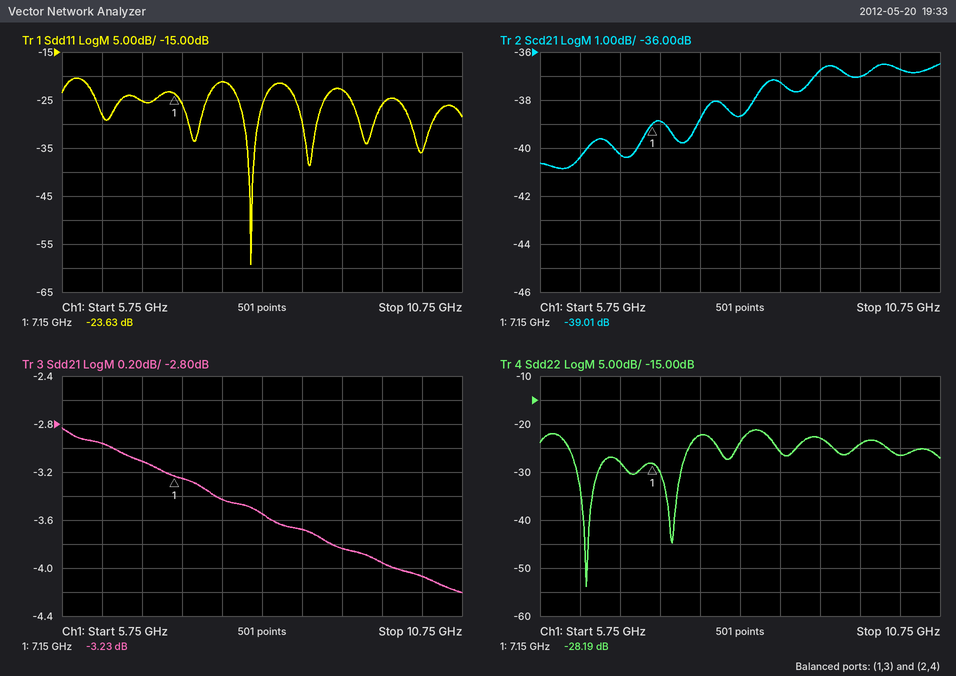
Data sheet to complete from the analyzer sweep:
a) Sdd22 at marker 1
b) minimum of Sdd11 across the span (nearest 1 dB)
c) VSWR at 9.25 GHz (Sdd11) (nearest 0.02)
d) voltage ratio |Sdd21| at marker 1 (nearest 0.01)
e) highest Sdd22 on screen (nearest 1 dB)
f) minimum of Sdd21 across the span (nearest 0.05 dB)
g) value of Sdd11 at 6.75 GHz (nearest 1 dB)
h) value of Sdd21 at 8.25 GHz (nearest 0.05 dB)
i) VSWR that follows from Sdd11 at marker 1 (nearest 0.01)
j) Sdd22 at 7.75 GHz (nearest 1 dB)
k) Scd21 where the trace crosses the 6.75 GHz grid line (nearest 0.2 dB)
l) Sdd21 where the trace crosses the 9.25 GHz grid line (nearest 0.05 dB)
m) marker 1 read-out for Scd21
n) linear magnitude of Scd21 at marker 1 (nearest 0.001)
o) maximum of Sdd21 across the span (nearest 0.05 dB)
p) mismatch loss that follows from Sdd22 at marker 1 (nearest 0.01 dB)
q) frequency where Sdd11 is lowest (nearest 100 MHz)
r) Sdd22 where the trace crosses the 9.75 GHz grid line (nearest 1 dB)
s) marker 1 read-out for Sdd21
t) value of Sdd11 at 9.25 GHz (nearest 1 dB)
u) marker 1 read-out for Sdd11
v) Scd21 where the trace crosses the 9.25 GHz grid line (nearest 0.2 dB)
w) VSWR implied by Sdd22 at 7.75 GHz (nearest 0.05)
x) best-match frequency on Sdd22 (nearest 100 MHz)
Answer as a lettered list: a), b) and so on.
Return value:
a) -28.19 dB
b) -59 dB
c) 1.16
d) 0.69
e) -21 dB
f) -4.20 dB
g) -25 dB
h) -3.55 dB
i) 1.14
j) -22 dB
k) -40.2 dB
l) -3.85 dB
m) -39.01 dB
n) 0.011
o) -2.85 dB
p) 0.01 dB
q) 8.1 GHz
r) -24 dB
s) -3.23 dB
t) -23 dB
u) -23.63 dB
v) -36.8 dB
w) 1.15
x) 6.3 GHz
